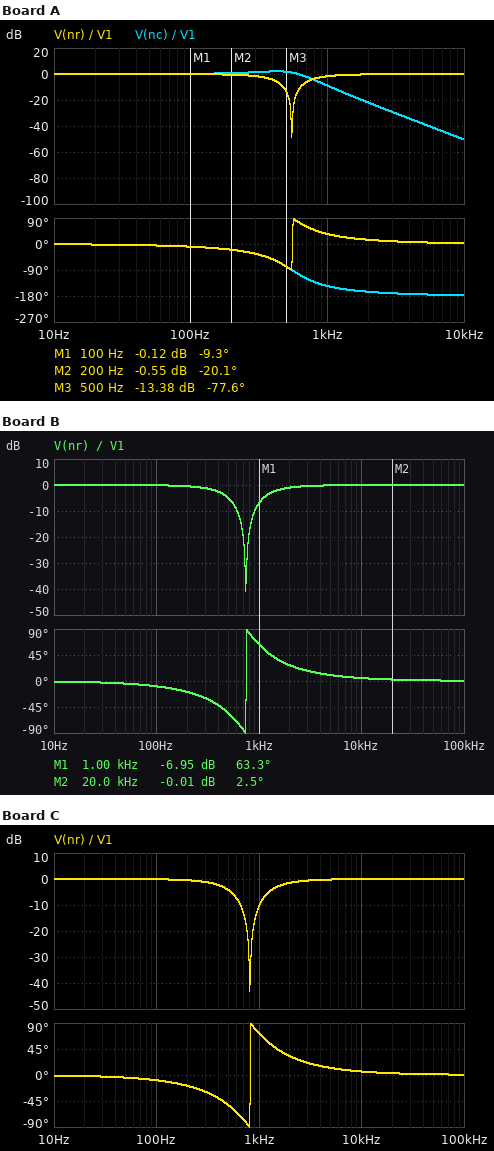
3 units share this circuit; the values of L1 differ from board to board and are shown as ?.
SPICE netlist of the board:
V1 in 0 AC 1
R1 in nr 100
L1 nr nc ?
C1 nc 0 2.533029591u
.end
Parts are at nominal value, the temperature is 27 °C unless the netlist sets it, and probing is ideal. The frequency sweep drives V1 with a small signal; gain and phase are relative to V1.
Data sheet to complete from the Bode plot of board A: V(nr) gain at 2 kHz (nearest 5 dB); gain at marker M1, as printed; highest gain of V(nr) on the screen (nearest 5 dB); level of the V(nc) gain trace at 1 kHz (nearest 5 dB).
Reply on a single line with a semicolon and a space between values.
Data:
0 dB; -0.12 dB; 0 dB; -10 dB
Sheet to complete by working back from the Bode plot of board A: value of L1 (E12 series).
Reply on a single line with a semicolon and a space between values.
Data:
33 mH
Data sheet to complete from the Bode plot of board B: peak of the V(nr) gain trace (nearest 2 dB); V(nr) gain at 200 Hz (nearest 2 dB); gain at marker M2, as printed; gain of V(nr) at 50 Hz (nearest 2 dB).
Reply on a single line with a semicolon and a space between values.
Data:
0 dB; 0 dB; -0.01 dB; 0 dB
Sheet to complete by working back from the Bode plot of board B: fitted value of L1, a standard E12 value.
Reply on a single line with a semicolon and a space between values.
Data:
18 mH
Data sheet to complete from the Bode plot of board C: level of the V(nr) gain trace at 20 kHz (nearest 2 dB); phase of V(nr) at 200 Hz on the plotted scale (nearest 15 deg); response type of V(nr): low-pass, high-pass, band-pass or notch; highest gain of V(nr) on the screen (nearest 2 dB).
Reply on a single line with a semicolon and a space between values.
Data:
0 dB; -15 deg; notch; 0 dB
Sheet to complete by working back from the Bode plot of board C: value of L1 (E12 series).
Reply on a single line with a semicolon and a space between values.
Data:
15 mH
